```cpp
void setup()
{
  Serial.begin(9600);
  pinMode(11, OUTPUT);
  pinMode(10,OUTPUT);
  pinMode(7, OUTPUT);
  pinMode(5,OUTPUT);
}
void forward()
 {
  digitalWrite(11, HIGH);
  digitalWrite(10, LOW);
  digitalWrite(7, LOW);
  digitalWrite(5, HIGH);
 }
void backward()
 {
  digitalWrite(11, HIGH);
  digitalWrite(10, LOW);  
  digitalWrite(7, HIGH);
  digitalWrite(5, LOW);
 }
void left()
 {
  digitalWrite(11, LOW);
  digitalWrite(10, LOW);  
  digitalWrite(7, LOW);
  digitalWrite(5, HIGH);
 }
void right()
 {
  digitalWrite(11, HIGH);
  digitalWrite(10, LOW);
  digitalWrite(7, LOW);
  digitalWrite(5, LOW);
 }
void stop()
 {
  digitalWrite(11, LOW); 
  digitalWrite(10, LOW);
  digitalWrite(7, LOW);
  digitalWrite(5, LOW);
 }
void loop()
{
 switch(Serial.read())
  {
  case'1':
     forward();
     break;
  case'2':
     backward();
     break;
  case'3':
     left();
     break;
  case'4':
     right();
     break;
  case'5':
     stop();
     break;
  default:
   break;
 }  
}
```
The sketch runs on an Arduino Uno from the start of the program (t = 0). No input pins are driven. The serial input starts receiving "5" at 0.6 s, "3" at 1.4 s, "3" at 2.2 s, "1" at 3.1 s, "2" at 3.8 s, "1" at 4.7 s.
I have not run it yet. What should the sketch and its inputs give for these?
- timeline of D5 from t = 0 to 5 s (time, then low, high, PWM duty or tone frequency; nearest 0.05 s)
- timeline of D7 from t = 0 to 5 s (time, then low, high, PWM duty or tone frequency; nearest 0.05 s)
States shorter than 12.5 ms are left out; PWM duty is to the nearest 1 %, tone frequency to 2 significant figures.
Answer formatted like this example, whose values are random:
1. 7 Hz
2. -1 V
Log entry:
1. 0 s low; 1.4 s high; 3.8 s low; 4.7 s high
2. 0 s low; 3.8 s high; 4.7 s low
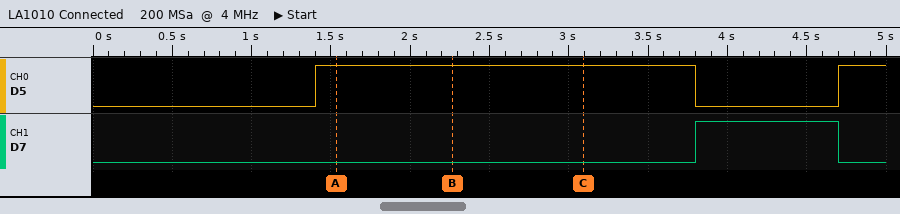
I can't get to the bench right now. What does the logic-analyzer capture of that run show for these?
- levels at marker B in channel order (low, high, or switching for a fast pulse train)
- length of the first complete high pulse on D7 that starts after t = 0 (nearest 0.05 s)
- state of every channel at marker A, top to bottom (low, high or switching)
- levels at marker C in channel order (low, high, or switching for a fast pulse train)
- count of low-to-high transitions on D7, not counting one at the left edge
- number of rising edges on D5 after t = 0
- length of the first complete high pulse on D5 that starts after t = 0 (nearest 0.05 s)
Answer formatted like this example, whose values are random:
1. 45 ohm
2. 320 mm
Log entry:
1. D5 high, D7 low
2. 0.90 s
3. D5 high, D7 low
4. D5 high, D7 low
5. 1
6. 2
7. 2.40 s
